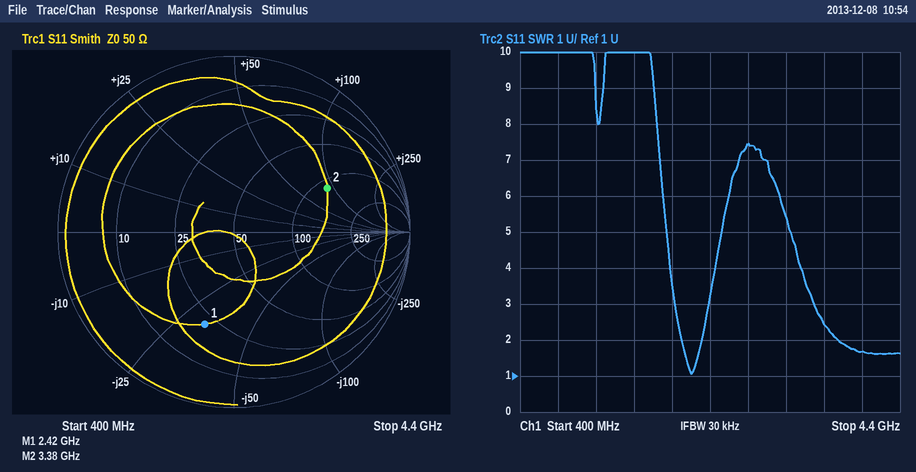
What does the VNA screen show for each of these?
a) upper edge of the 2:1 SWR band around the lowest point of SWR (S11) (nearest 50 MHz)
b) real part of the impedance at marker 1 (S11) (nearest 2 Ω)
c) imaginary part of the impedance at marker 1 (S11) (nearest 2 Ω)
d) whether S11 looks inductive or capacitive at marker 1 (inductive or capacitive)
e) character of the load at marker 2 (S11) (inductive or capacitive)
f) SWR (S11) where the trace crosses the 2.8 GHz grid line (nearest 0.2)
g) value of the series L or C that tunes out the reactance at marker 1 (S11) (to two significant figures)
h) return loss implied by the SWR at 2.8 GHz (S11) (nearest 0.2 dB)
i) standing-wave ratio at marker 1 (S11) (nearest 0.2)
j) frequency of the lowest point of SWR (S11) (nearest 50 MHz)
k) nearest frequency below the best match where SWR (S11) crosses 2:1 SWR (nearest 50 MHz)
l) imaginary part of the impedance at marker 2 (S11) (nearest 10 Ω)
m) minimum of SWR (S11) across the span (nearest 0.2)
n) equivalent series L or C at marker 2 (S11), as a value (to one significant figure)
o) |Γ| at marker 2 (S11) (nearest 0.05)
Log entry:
2.30 GHz
22 Ω
-32 Ω
capacitive
inductive
7.4
2.1 nH
2.4 dB
3.4
2.20 GHz
2.10 GHz
+90 Ω
1.0
4 nH
0.60
